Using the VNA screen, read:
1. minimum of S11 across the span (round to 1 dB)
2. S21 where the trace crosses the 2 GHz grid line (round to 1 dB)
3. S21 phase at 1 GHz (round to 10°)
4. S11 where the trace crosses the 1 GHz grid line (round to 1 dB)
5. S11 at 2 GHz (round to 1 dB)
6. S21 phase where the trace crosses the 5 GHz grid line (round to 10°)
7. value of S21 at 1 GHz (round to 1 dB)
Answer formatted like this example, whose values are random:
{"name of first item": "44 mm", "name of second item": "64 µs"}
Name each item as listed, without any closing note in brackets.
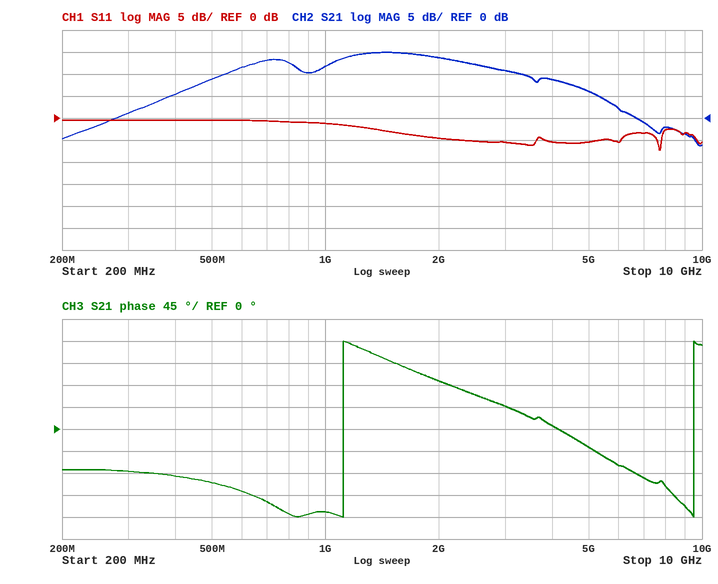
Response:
{"minimum of S11 across the span": "-7 dB", "S21 where the trace crosses the 2 GHz grid line": "14 dB", "S21 phase at 1 GHz": "-170°", "S11 where the trace crosses the 1 GHz grid line": "-1 dB", "S11 at 2 GHz": "-5 dB", "S21 phase where the trace crosses the 5 GHz grid line": "-40°", "value of S21 at 1 GHz": "12 dB"}
